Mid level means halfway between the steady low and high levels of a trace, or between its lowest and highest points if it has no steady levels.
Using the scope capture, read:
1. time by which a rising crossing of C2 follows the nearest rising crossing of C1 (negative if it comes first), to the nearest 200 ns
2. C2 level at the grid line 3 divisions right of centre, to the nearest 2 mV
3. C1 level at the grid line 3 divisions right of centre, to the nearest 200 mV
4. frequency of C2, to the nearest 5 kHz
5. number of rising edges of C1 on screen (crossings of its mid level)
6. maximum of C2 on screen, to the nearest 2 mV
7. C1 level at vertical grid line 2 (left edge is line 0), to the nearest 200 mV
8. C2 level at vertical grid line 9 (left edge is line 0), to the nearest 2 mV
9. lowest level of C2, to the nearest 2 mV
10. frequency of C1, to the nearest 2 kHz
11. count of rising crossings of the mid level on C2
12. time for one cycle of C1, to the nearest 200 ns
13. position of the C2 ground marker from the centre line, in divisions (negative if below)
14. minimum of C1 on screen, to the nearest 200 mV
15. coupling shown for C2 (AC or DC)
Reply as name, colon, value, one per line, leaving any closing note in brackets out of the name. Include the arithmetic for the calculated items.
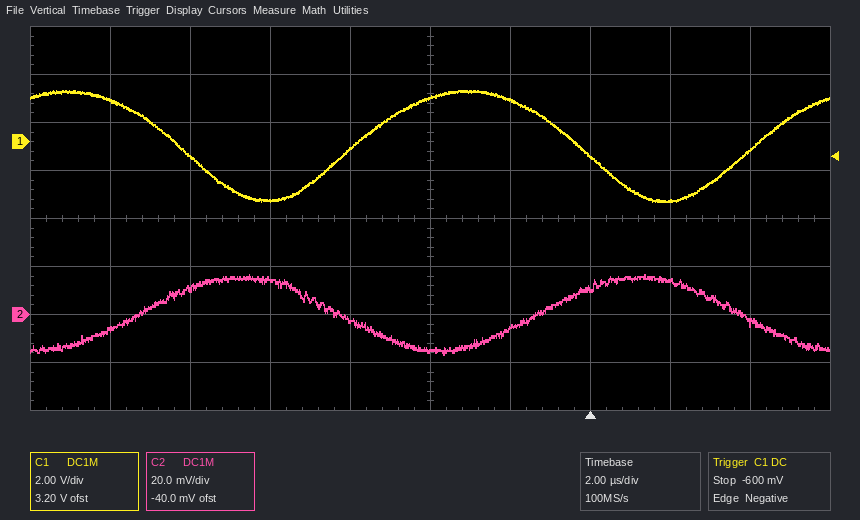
time by which a rising crossing of C2 follows the nearest rising crossing of C1 (negative if it comes first), to the nearest 200 ns: +4.6 µs
C2 level at the grid line 3 divisions right of centre, to the nearest 2 mV: 14 mV
C1 level at the grid line 3 divisions right of centre, to the nearest 200 mV: -2.4 V
frequency of C2, to the nearest 5 kHz: 100 kHz
number of rising edges of C1 on screen: 2
maximum of C2 on screen, to the nearest 2 mV: 16 mV
C1 level at vertical grid line 2 (left edge is line 0), to the nearest 200 mV: -600 mV
C2 level at vertical grid line 9 (left edge is line 0), to the nearest 2 mV: -2 mV
lowest level of C2, to the nearest 2 mV: -16 mV
frequency of C1, to the nearest 2 kHz: 1 / 10.0 µs ≈ 100 kHz
count of rising crossings of the mid level on C2: 2
time for one cycle of C1, to the nearest 200 ns: 10.0 µs
position of the C2 ground marker from the centre line, in divisions: -2.0 div
minimum of C1 on screen, to the nearest 200 mV: -2.4 V
coupling shown for C2: DC
